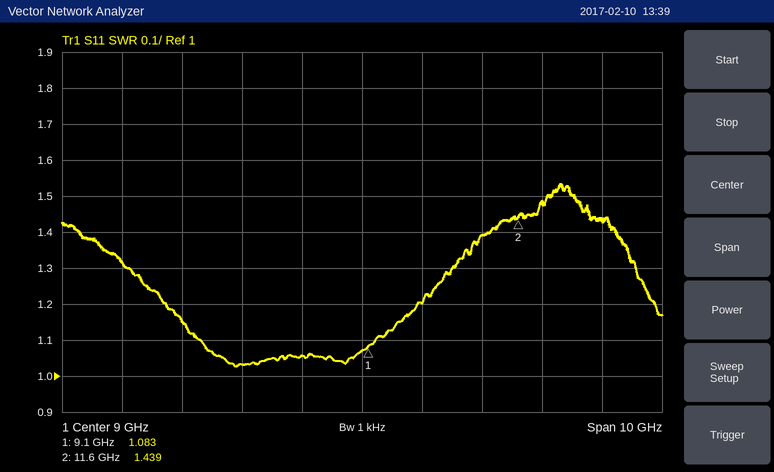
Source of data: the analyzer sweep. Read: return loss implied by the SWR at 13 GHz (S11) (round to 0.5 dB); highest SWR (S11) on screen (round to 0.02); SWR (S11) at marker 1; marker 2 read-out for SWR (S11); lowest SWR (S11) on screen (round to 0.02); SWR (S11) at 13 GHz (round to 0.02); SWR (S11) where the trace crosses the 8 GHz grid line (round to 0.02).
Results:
15.0 dB
1.54
1.083
1.439
1.02
1.44
1.06
